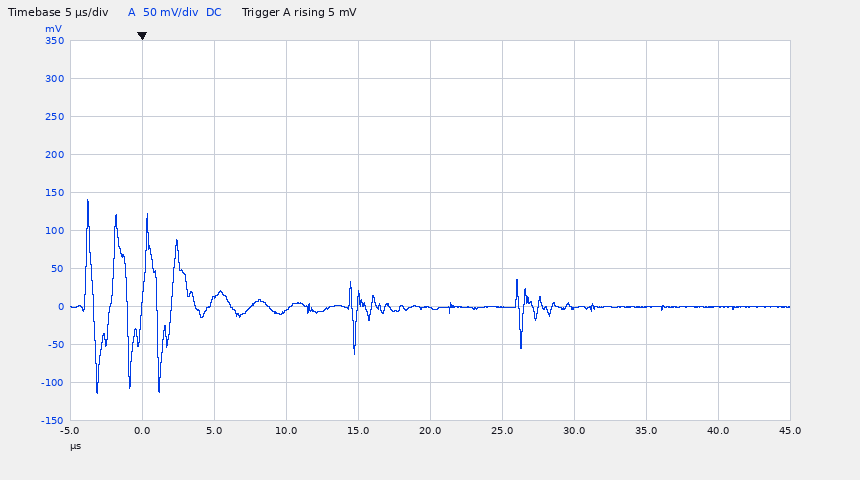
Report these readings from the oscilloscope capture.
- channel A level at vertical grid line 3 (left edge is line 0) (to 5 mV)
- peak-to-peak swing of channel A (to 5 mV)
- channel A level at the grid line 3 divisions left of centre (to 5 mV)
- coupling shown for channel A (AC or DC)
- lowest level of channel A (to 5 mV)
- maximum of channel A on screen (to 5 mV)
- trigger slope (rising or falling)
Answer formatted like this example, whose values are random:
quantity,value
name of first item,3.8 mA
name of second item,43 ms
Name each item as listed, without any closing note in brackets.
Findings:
quantity,value
channel A level at vertical grid line 3 (left edge is line 0),-5 mV
peak-to-peak swing of channel A,255 mV
channel A level at the grid line 3 divisions left of centre,10 mV
coupling shown for channel A,DC
lowest level of channel A,-115 mV
maximum of channel A on screen,140 mV
trigger slope,rising
